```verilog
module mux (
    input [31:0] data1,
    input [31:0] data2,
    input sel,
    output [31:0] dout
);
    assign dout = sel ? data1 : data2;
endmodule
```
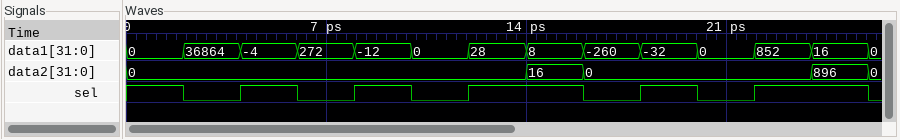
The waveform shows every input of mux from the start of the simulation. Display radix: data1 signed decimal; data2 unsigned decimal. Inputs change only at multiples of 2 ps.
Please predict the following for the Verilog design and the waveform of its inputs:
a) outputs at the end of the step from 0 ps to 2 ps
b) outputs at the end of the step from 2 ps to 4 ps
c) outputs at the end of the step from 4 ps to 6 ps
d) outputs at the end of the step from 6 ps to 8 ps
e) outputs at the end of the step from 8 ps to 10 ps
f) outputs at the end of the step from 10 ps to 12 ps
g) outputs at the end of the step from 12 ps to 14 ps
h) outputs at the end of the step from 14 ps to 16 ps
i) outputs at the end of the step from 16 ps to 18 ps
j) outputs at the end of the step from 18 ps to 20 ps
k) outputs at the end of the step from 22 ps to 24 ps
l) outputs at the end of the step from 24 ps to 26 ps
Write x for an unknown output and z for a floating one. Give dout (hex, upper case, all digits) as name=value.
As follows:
dout=00000000
dout=00000000
dout=FFFFFFFC
dout=00000000
dout=FFFFFFF4
dout=00000000
dout=0000001C
dout=00000008
dout=00000000
dout=FFFFFFE0
dout=00000354
dout=00000010
